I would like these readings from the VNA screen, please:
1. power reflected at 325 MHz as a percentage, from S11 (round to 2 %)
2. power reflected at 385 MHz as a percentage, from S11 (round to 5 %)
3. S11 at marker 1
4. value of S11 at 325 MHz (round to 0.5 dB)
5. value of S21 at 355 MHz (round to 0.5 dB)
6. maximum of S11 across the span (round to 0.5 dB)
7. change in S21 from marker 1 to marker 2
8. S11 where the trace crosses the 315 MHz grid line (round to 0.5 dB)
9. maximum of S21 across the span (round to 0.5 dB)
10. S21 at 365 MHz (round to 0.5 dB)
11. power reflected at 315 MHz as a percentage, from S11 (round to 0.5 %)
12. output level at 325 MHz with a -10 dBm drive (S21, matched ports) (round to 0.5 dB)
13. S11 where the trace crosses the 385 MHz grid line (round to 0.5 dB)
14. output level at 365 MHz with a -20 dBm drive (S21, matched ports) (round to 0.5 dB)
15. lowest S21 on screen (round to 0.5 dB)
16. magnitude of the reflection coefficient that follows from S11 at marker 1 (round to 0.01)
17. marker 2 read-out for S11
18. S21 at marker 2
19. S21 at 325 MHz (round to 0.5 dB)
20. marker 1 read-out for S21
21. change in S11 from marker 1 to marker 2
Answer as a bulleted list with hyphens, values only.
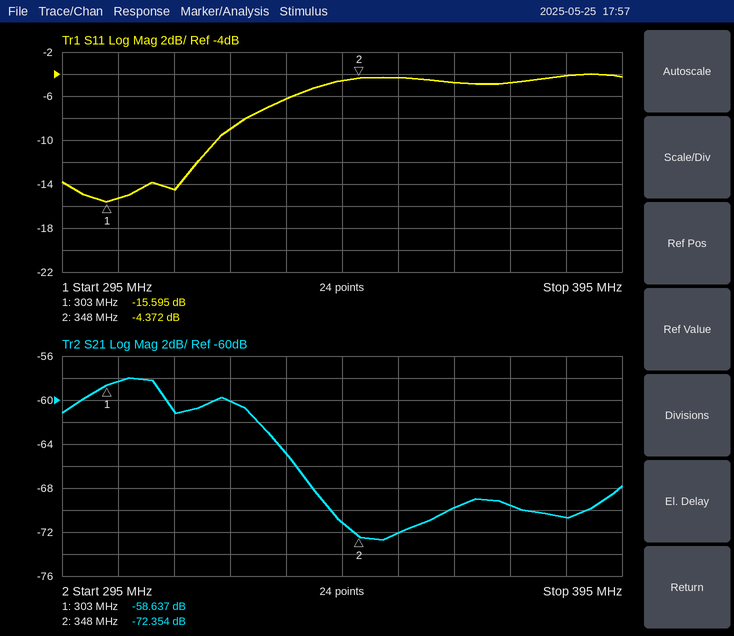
- 12 %
- 40 %
- -15.595 dB
- -9.0 dB
- -72.0 dB
- -4.0 dB
- -13.717 dB
- -14.5 dB
- -58.0 dB
- -70.0 dB
- 3.5 %
- -70.0 dBm
- -4.0 dB
- -90.0 dBm
- -72.5 dB
- 0.17
- -4.372 dB
- -72.354 dB
- -60.0 dB
- -58.637 dB
- 11.223 dB
